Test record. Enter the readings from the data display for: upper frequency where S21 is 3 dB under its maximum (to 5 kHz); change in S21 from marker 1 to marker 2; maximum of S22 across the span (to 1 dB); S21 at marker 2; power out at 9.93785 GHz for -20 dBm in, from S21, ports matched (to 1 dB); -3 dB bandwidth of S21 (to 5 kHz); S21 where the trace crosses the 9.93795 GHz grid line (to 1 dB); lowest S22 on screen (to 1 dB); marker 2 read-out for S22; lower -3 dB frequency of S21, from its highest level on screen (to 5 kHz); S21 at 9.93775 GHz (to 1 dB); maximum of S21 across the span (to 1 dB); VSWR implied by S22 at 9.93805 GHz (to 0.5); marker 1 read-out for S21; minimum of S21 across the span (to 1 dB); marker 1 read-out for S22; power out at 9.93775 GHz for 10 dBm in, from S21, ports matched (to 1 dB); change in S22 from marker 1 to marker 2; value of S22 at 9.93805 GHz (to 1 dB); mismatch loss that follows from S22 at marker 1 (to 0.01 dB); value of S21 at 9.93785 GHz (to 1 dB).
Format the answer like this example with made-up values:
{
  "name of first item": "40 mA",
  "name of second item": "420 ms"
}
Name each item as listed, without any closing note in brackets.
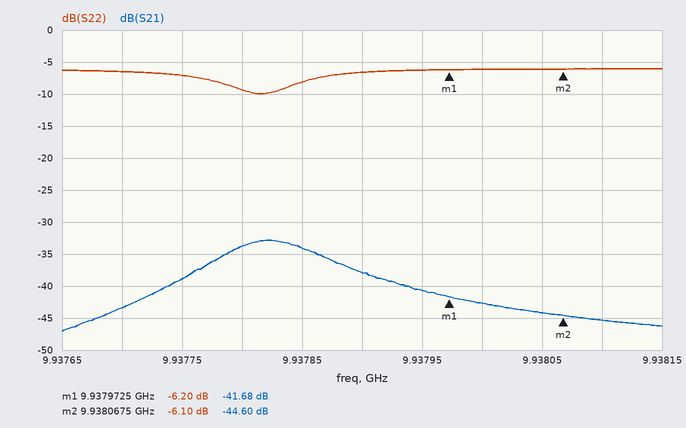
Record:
{
  "upper frequency where S21 is 3 dB under its maximum": "9.937875 GHz",
  "change in S21 from marker 1 to marker 2": "-2.92 dB",
  "maximum of S22 across the span": "-6 dB",
  "S21 at marker 2": "-44.60 dB",
  "power out at 9.93785 GHz for -20 dBm in, from S21, ports matched": "-54 dBm",
  "-3 dB bandwidth of S21": "95 kHz",
  "S21 where the trace crosses the 9.93795 GHz grid line": "-41 dB",
  "lowest S22 on screen": "-10 dB",
  "marker 2 read-out for S22": "-6.10 dB",
  "lower -3 dB frequency of S21, from its highest level on screen": "9.937780 GHz",
  "S21 at 9.93775 GHz": "-39 dB",
  "maximum of S21 across the span": "-33 dB",
  "VSWR implied by S22 at 9.93805 GHz": "3.0",
  "marker 1 read-out for S21": "-41.68 dB",
  "minimum of S21 across the span": "-47 dB",
  "marker 1 read-out for S22": "-6.20 dB",
  "power out at 9.93775 GHz for 10 dBm in, from S21, ports matched": "-29 dBm",
  "change in S22 from marker 1 to marker 2": "0.10 dB",
  "value of S22 at 9.93805 GHz": "-6 dB",
  "mismatch loss that follows from S22 at marker 1": "1.19 dB",
  "value of S21 at 9.93785 GHz": "-34 dB"
}
